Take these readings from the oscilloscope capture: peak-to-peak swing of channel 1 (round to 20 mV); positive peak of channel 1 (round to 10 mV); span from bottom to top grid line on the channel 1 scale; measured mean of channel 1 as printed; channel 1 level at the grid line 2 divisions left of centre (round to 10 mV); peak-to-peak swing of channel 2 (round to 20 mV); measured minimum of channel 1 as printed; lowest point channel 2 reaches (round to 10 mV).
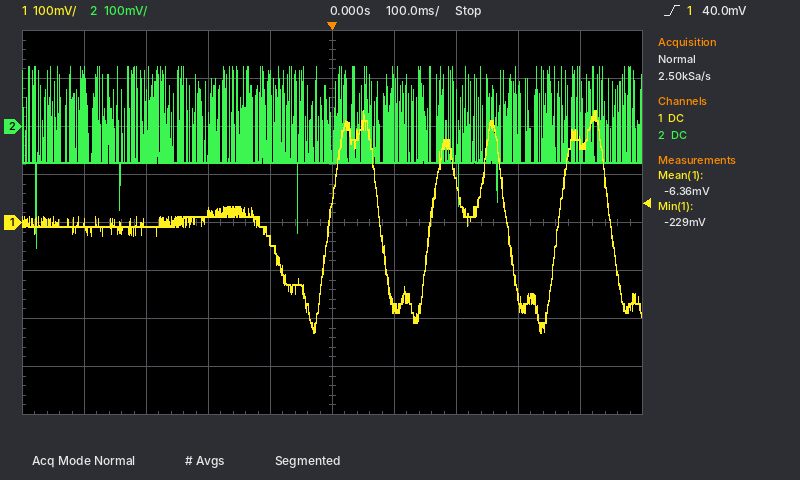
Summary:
460 mV
230 mV
800 mV
-6.36 mV
20 mV
380 mV
-229 mV
-250 mV
